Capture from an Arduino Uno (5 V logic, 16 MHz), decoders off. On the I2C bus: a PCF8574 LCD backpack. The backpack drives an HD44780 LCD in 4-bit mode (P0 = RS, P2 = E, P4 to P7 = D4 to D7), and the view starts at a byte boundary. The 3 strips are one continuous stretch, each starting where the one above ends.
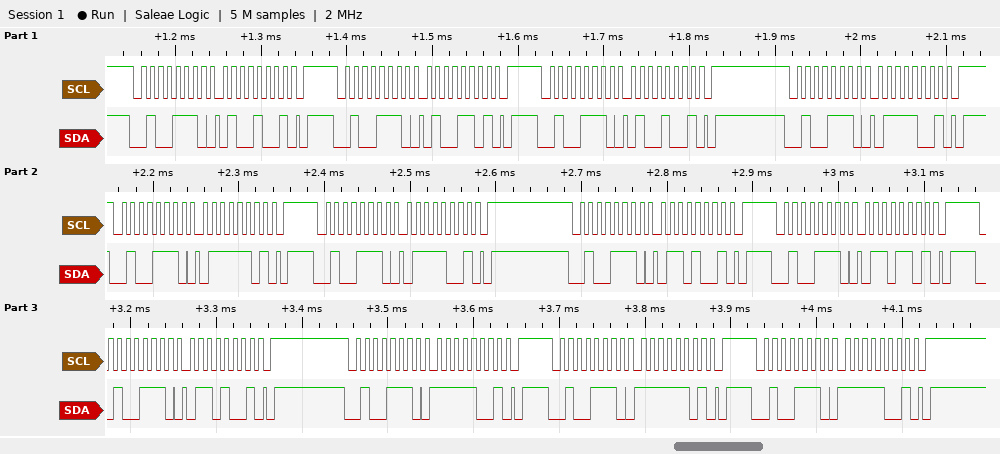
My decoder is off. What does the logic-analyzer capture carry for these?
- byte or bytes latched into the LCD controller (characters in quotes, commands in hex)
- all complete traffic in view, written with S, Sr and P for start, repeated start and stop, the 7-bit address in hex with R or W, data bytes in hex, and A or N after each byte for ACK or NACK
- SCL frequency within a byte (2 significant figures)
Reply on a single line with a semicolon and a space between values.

'G' 'o'; S 27W A 49 A P S 27W A 4D A P S 27W A 49 A P S 27W A 79 A P S 27W A 7D A P S 27W A 79 A P S 27W A 69 A P S 27W A 6D A P S 27W A 69 A P S 27W A F9 A P S 27W A FD A P S 27W A F9 A P; 100 kHz
